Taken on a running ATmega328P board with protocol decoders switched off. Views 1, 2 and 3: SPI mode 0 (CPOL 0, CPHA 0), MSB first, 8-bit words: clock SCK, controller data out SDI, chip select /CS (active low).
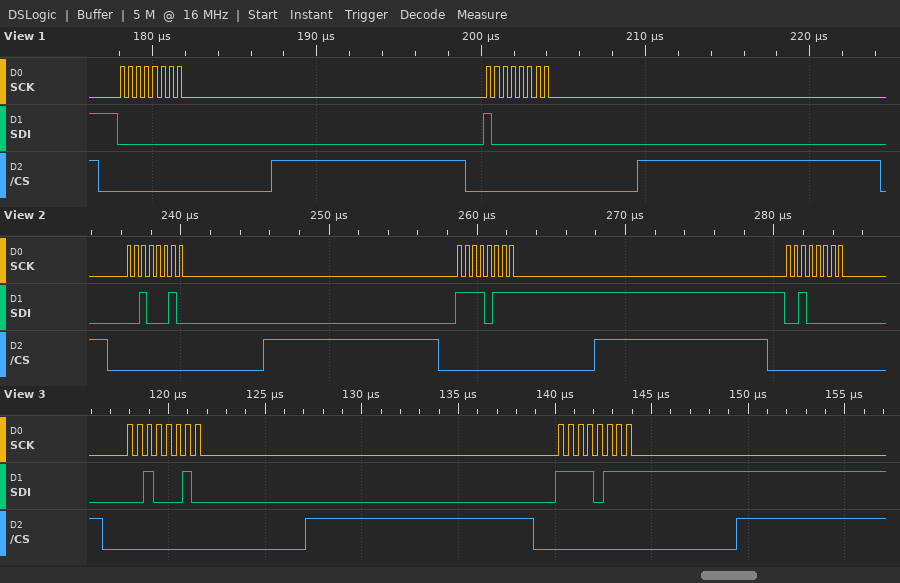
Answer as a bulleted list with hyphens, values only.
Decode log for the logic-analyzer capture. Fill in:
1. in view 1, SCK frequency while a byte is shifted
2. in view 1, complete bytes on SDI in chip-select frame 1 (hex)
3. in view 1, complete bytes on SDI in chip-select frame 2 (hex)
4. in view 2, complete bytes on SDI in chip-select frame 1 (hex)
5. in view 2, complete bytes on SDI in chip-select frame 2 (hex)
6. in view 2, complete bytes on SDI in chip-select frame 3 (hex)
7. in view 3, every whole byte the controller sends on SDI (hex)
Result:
- 2 MHz
- 0x00
- 0x80
- 22
- F7
- 20
- 22 F7
